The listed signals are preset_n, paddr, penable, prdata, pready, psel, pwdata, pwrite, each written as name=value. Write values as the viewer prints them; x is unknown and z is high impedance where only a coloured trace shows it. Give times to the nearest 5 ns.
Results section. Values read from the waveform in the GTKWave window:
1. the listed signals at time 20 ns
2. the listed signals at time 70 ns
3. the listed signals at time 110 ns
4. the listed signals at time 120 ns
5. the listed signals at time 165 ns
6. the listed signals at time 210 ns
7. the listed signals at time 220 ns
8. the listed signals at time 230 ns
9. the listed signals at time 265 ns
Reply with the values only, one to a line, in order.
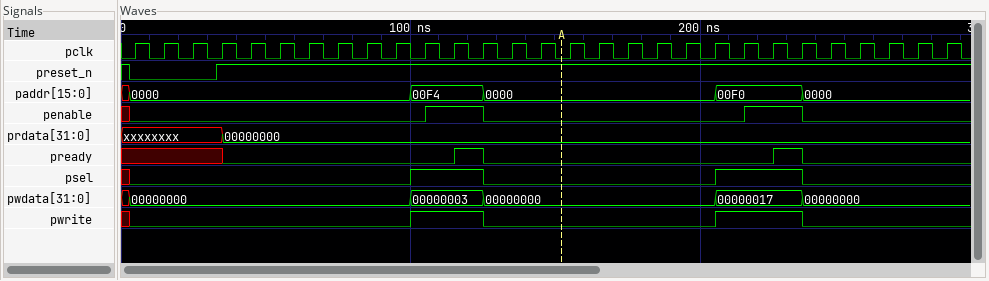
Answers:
preset_n=0, paddr=0000, penable=0, prdata=xxxxxxxx, pready=x, psel=0, pwdata=00000000, pwrite=0
preset_n=1, paddr=0000, penable=0, prdata=00000000, pready=0, psel=0, pwdata=00000000, pwrite=0
preset_n=1, paddr=00F4, penable=1, prdata=00000000, pready=0, psel=1, pwdata=00000003, pwrite=1
preset_n=1, paddr=00F4, penable=1, prdata=00000000, pready=1, psel=1, pwdata=00000003, pwrite=1
preset_n=1, paddr=0000, penable=0, prdata=00000000, pready=0, psel=0, pwdata=00000000, pwrite=0
preset_n=1, paddr=00F0, penable=0, prdata=00000000, pready=0, psel=1, pwdata=00000017, pwrite=1
preset_n=1, paddr=00F0, penable=1, prdata=00000000, pready=0, psel=1, pwdata=00000017, pwrite=1
preset_n=1, paddr=00F0, penable=1, prdata=00000000, pready=1, psel=1, pwdata=00000017, pwrite=1
preset_n=1, paddr=0000, penable=0, prdata=00000000, pready=0, psel=0, pwdata=00000000, pwrite=0
